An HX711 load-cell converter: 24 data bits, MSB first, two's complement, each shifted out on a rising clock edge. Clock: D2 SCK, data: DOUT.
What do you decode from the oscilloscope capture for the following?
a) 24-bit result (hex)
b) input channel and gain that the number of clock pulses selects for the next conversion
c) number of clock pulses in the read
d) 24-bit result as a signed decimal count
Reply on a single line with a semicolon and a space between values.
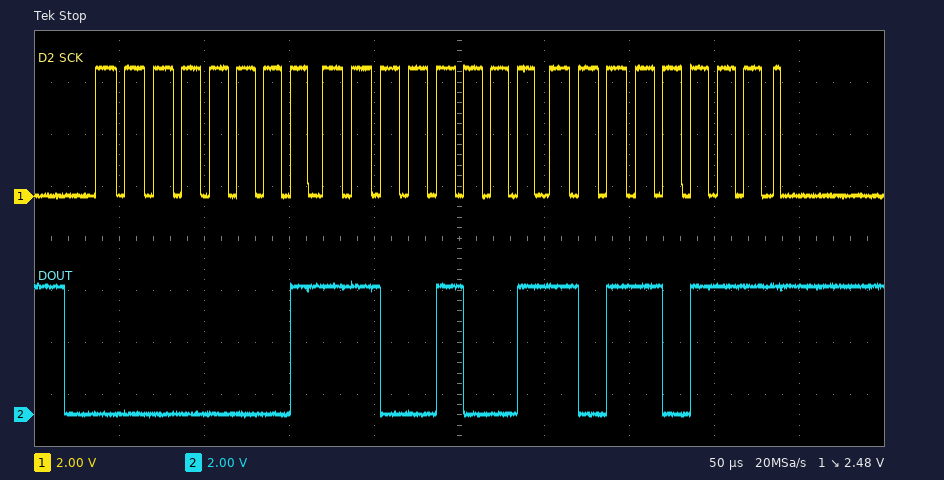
0x01C9B7; channel A, gain 128; 25; 117175
